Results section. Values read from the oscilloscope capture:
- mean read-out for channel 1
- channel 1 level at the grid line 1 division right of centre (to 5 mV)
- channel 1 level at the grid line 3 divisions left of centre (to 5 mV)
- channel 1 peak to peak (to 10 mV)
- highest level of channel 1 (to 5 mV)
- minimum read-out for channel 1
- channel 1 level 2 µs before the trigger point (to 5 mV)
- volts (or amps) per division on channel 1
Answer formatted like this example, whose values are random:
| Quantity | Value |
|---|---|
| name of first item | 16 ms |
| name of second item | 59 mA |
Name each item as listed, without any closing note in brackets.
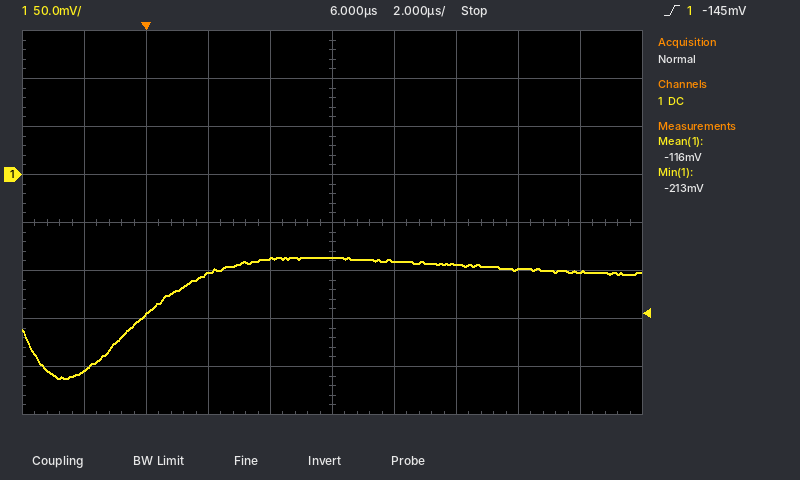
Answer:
| Quantity | Value |
|---|---|
| mean read-out for channel 1 | -116 mV |
| channel 1 level at the grid line 1 division right of centre | -90 mV |
| channel 1 level at the grid line 3 divisions left of centre | -145 mV |
| channel 1 peak to peak | 130 mV |
| highest level of channel 1 | -85 mV |
| minimum read-out for channel 1 | -213 mV |
| channel 1 level 2 µs before the trigger point | -205 mV |
| volts (or amps) per division on channel 1 | 50 mV |
